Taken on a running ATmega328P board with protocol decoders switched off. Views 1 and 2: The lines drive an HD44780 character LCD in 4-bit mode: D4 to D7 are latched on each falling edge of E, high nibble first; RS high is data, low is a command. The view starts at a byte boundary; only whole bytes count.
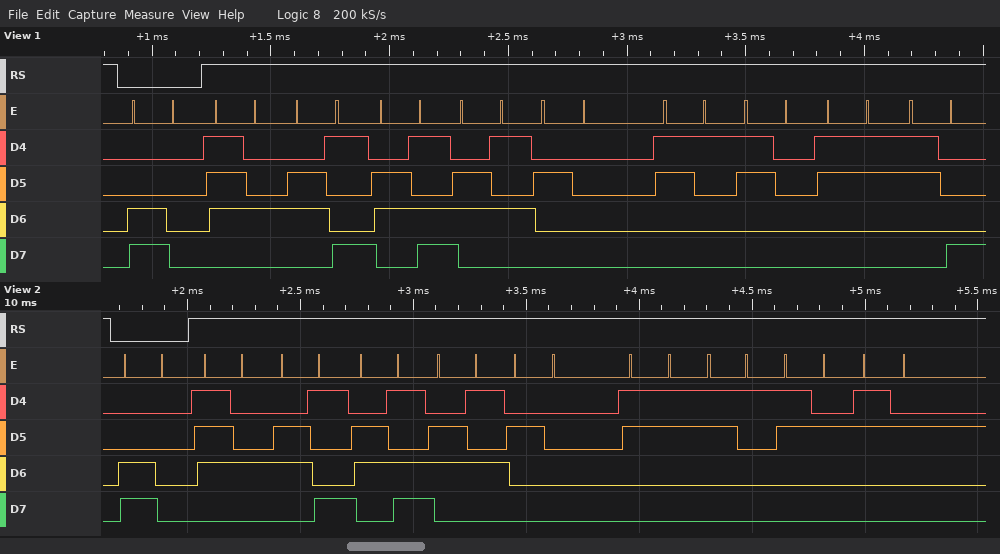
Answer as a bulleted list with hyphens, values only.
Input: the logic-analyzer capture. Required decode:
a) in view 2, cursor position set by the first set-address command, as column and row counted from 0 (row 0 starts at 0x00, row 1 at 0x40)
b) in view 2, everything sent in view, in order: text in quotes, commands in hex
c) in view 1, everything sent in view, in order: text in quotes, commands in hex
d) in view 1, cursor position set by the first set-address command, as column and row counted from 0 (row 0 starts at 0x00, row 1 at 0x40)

- column 0, row 1
- 0xC0 "time 3122"
- 0xC0 "time 1038"
- column 0, row 1
